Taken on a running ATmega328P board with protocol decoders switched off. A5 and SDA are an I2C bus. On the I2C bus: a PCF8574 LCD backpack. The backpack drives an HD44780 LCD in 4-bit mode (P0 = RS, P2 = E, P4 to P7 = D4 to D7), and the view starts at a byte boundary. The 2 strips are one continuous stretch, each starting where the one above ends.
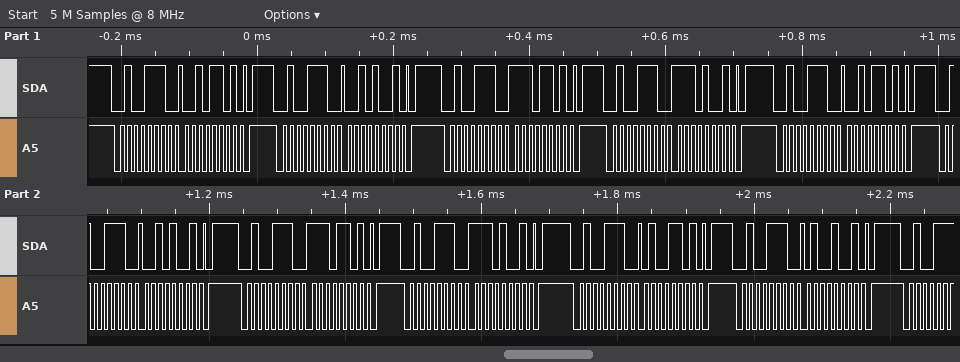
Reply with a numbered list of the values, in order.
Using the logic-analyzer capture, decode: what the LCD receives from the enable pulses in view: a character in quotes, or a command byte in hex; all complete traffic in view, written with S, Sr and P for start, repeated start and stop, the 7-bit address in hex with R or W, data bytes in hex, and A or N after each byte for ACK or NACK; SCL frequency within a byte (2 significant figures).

1. '.' '.'
2. S 27W A 2D A P S 27W A 29 A P S 27W A ED A P S 27W A E9 A P S 27W A 2D A P S 27W A 29 A P S 27W A ED A P S 27W A E9 A P S 27W A 4D A P S 27W A 49 A P
3. 100 kHz
